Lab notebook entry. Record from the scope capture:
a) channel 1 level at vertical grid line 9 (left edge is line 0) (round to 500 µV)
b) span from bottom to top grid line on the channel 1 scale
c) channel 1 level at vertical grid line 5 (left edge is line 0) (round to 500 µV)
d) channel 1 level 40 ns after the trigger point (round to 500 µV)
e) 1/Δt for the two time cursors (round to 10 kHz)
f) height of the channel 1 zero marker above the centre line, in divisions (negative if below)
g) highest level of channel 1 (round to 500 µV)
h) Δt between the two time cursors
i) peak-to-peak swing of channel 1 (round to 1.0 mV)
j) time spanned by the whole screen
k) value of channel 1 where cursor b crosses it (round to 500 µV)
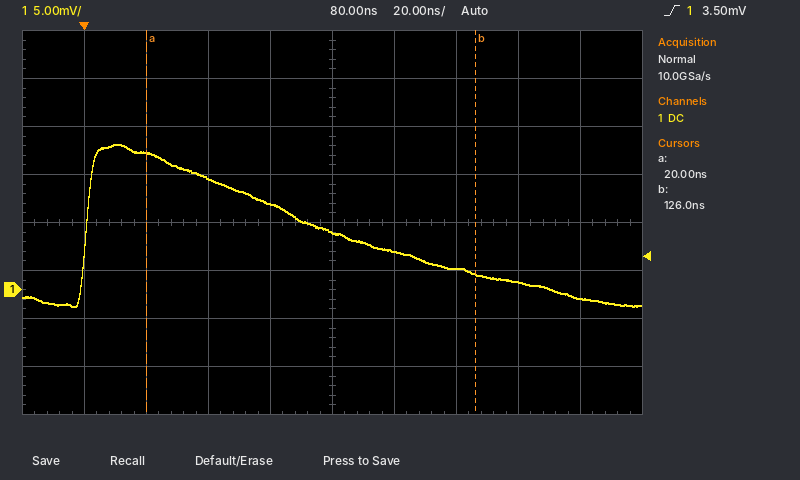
-1.0 mV
40 mV
6.0 mV
11.5 mV
9.43 MHz
-1.4 div
15.0 mV
106 ns
17.0 mV
200 ns
1.5 mV
